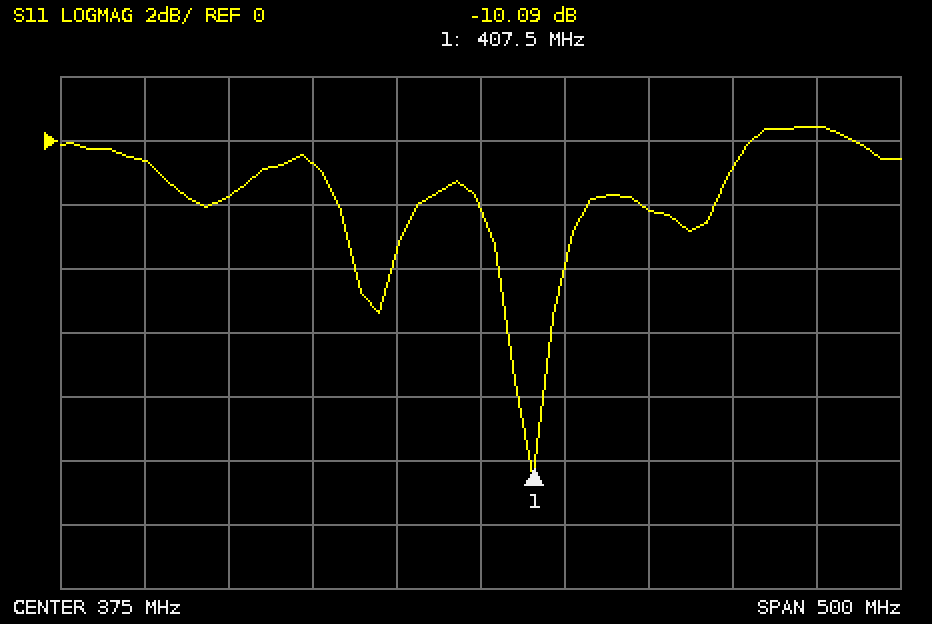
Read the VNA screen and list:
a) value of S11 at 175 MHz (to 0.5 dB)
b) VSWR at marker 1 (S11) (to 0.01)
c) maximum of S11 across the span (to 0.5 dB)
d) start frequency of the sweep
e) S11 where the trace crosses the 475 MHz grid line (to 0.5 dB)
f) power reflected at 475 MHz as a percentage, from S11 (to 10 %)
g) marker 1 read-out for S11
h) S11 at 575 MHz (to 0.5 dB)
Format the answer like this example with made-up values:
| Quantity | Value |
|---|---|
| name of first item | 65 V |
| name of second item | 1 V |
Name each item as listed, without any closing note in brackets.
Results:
| Quantity | Value |
|---|---|
| value of S11 at 175 MHz | -0.5 dB |
| VSWR at marker 1 (S11) | 1.91 |
| maximum of S11 across the span | 0.5 dB |
| start frequency of the sweep | 125 MHz |
| S11 where the trace crosses the 475 MHz grid line | -2.0 dB |
| power reflected at 475 MHz as a percentage, from S11 | 60 % |
| marker 1 read-out for S11 | -10.09 dB |
| S11 at 575 MHz | 0.5 dB |
